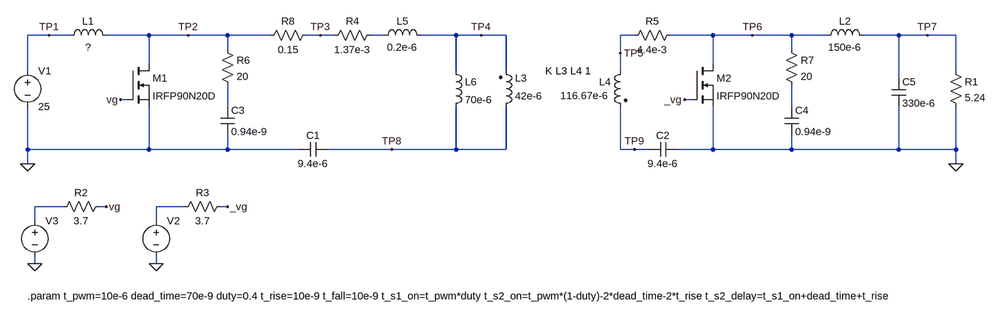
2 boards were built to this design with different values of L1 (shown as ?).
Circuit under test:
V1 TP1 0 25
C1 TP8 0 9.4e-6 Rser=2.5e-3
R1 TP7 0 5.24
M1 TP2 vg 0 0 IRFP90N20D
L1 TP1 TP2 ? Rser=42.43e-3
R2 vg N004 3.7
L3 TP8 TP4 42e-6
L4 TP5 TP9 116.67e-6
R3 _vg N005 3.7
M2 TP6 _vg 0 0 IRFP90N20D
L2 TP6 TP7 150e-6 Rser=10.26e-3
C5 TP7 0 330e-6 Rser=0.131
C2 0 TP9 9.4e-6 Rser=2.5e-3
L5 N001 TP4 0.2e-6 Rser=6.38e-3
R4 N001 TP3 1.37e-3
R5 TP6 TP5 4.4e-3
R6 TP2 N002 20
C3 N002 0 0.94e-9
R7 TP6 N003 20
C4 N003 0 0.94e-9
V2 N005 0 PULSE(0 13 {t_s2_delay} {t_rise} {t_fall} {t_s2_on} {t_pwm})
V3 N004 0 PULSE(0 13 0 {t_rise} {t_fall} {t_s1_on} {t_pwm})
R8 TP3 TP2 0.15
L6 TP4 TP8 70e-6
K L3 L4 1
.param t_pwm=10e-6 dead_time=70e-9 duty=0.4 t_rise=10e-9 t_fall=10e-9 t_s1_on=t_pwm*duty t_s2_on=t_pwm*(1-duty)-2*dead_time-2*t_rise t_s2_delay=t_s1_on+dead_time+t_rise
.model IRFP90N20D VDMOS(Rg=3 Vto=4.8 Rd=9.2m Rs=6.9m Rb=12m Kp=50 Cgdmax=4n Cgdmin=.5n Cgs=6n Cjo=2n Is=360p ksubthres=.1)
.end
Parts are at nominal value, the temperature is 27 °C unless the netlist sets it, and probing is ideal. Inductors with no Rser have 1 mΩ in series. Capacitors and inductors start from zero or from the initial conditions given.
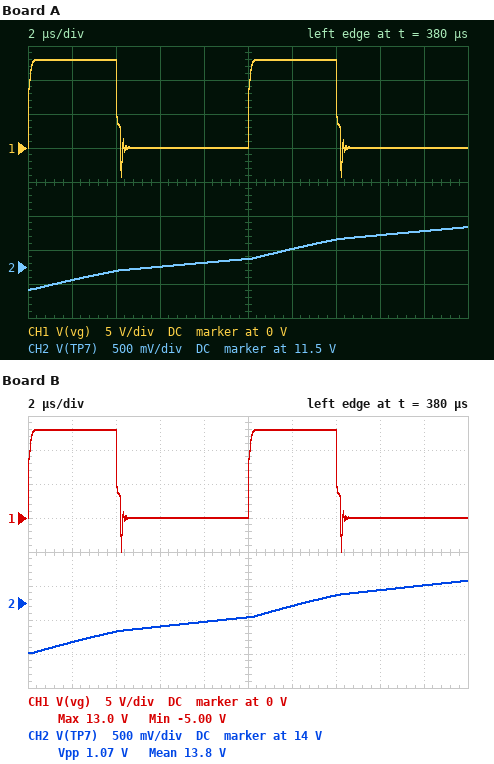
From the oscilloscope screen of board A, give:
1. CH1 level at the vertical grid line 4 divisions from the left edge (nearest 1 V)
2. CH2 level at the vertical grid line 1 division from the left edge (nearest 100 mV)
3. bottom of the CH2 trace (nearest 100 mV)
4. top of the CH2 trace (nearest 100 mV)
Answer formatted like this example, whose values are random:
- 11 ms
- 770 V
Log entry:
- 0 V
- 11.3 V
- 11.2 V
- 12.1 V
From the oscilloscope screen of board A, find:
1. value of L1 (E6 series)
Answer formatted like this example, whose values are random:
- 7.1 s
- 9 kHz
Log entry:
- 220 µH
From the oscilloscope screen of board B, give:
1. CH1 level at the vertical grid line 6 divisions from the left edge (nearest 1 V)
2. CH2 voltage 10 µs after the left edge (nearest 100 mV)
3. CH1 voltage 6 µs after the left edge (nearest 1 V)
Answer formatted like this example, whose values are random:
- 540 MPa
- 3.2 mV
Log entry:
- 13 V
- 13.8 V
- 0 V
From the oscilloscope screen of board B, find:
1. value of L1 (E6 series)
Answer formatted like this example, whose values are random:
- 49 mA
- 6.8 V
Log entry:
- 150 µH
